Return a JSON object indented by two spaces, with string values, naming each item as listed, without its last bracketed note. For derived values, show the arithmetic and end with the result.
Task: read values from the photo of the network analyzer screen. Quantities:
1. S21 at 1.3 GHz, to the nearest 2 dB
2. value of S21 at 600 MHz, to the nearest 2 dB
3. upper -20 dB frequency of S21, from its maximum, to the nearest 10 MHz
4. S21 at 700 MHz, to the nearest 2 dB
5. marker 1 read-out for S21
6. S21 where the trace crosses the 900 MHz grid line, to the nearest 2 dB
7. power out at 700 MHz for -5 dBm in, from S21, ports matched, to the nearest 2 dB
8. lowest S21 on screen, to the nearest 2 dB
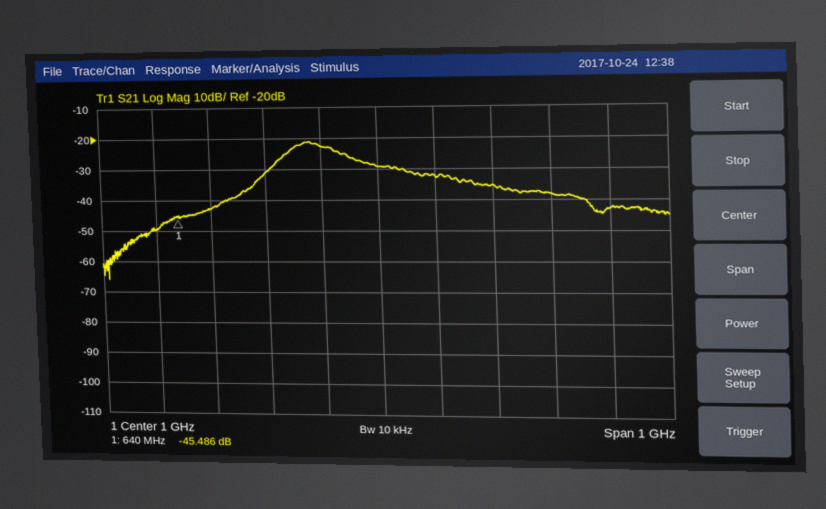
{
  "S21 at 1.3 GHz, to the nearest 2 dB": "-38 dB",
  "value of S21 at 600 MHz, to the nearest 2 dB": "-50 dB",
  "upper -20 dB frequency of S21, from its maximum, to the nearest 10 MHz": "1.36 GHz",
  "S21 at 700 MHz, to the nearest 2 dB": "-42 dB",
  "marker 1 read-out for S21": "-45.486 dB",
  "S21 where the trace crosses the 900 MHz grid line, to the nearest 2 dB": "-22 dB",
  "power out at 700 MHz for -5 dBm in, from S21, ports matched, to the nearest 2 dB": "-5 dBm + (-42 dB) = -48 dBm",
  "lowest S21 on screen, to the nearest 2 dB": "-66 dB"
}
